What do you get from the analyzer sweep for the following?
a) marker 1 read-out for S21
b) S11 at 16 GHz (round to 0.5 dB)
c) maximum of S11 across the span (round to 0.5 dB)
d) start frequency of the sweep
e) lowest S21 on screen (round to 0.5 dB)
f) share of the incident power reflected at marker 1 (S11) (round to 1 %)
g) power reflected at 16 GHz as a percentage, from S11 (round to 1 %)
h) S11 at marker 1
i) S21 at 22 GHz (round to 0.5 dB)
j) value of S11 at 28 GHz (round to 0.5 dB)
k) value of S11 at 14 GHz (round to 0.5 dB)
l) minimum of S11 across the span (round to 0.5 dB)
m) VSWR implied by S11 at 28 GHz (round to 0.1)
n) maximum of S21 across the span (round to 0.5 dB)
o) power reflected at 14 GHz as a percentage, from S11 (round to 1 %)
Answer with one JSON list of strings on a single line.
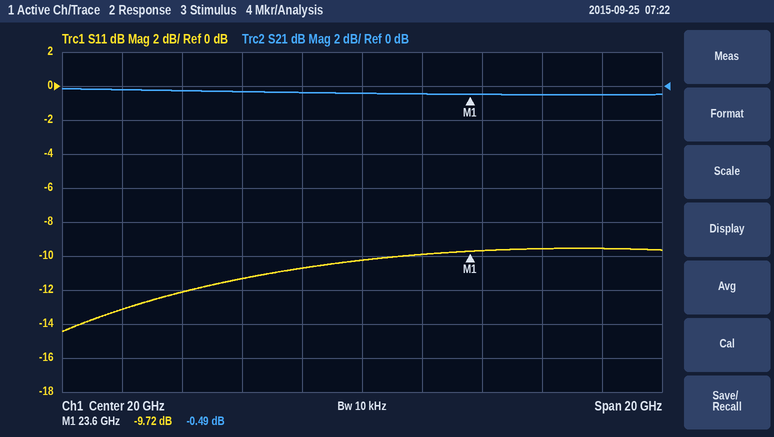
["-0.49 dB", "-11.5 dB", "-9.5 dB", "10 GHz", "-0.5 dB", "11 %", "7 %", "-9.72 dB", "-0.5 dB", "-9.5 dB", "-12.0 dB", "-14.5 dB", "2.0", "0.0 dB", "6 %"]
